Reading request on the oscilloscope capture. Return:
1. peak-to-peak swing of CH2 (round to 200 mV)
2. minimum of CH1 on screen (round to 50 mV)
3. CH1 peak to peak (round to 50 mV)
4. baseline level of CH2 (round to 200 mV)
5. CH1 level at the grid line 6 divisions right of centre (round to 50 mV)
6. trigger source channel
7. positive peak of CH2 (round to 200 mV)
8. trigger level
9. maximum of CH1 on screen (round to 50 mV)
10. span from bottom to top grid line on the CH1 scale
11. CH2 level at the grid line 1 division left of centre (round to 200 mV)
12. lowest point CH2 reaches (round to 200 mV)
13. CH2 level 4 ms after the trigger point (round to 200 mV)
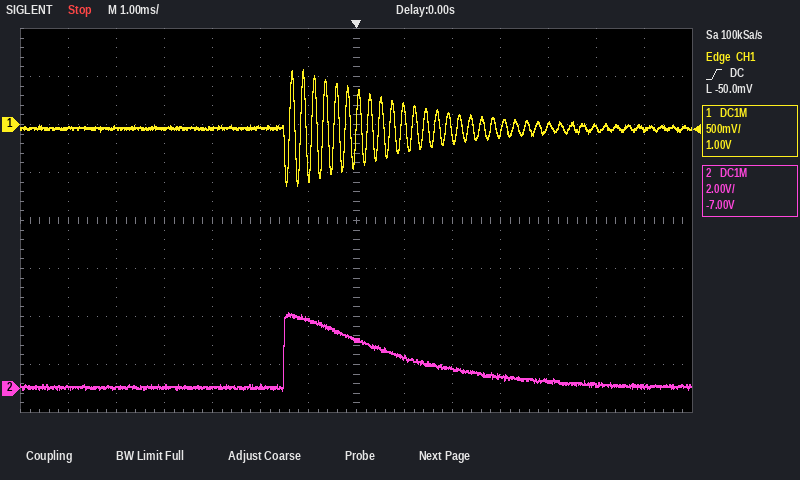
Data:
3.2 V
-650 mV
1.20 V
0.0 V
-50 mV
CH1
3.2 V
-50.0 mV
550 mV
4 V
2.8 V
0.0 V
400 mV
